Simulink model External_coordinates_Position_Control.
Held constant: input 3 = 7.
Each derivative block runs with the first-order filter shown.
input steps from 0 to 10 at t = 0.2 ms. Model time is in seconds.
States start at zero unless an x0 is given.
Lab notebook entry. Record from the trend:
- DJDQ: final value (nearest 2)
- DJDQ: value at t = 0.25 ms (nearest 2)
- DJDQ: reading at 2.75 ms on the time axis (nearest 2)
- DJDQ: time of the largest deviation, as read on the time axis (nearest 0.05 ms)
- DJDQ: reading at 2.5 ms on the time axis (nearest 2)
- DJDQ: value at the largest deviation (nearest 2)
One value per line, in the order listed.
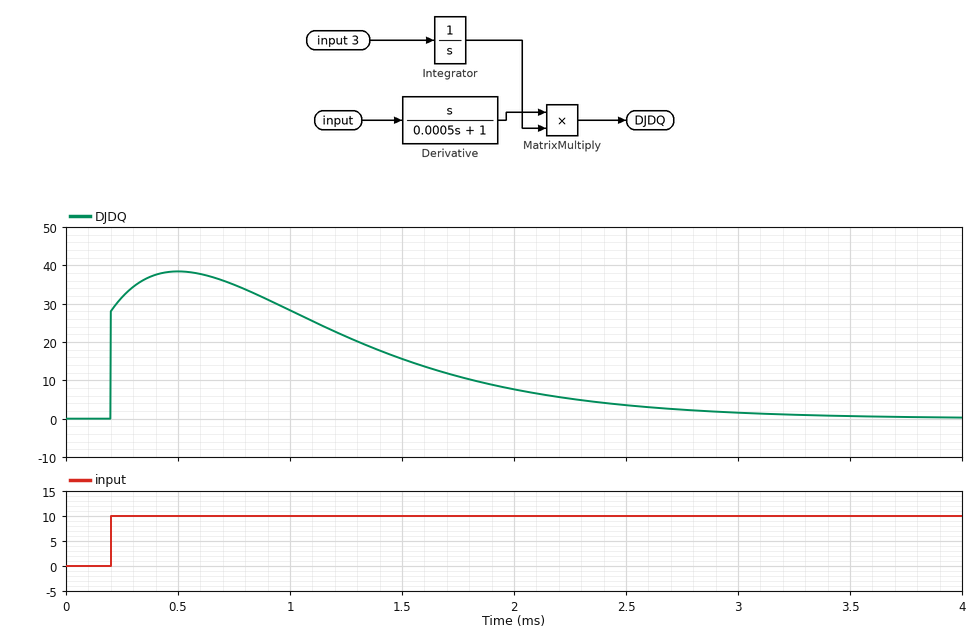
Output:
0
32
2
0.50 ms
4
38
